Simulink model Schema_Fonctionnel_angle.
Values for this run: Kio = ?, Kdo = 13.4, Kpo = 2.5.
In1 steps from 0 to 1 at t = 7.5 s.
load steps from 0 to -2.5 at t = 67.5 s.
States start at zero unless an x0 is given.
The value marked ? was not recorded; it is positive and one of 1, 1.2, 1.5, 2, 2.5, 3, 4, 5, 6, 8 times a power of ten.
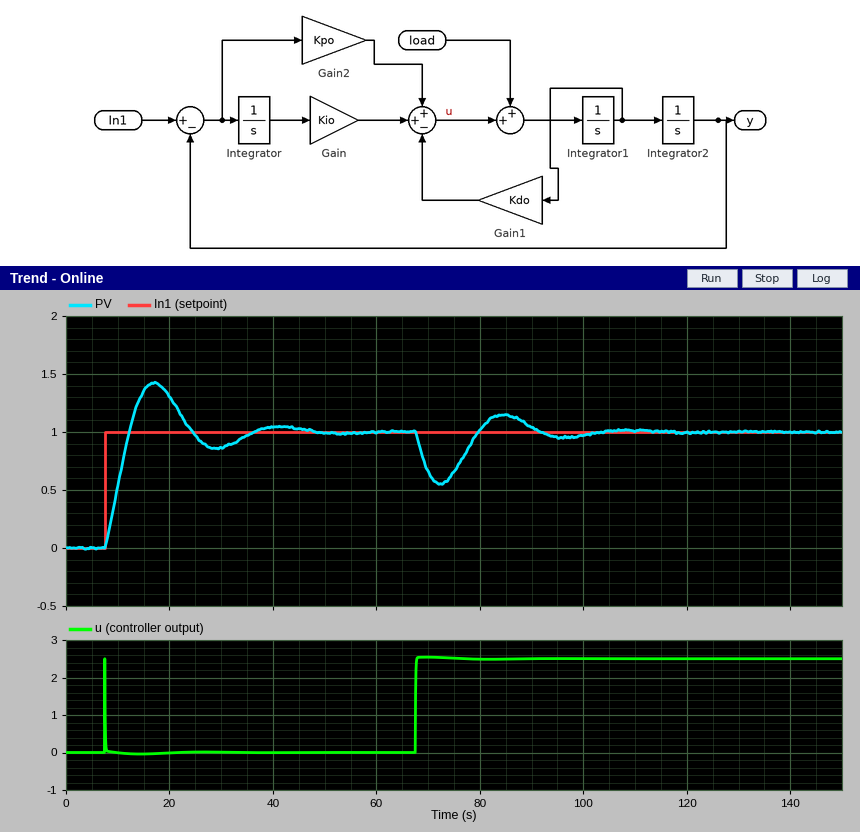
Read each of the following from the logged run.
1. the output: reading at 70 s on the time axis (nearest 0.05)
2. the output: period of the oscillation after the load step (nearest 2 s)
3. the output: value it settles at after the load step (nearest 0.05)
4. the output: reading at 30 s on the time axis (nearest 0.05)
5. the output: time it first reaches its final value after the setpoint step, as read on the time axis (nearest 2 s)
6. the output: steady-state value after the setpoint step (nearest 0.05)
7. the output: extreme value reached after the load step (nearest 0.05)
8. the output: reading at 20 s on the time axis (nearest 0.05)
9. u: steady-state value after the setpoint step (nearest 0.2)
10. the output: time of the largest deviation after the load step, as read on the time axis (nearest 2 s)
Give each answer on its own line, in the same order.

0.65
24 s
1.00
0.85
12 s
1.00
0.55
1.30
0.0
72 s
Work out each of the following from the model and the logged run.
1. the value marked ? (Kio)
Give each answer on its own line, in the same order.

1
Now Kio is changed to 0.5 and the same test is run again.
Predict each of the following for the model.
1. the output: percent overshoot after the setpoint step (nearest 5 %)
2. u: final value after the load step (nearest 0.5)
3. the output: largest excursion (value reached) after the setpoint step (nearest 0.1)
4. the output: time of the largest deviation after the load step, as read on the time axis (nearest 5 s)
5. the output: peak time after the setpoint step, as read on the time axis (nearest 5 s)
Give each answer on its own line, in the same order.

30 %
2.5
1.3
75 s
20 s
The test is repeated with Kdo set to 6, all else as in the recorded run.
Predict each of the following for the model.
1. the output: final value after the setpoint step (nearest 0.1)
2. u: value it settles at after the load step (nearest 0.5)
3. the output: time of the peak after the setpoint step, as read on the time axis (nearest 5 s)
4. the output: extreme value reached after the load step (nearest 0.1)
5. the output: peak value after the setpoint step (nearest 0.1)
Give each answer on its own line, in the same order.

1.0
2.5
15 s
0.4
1.3
